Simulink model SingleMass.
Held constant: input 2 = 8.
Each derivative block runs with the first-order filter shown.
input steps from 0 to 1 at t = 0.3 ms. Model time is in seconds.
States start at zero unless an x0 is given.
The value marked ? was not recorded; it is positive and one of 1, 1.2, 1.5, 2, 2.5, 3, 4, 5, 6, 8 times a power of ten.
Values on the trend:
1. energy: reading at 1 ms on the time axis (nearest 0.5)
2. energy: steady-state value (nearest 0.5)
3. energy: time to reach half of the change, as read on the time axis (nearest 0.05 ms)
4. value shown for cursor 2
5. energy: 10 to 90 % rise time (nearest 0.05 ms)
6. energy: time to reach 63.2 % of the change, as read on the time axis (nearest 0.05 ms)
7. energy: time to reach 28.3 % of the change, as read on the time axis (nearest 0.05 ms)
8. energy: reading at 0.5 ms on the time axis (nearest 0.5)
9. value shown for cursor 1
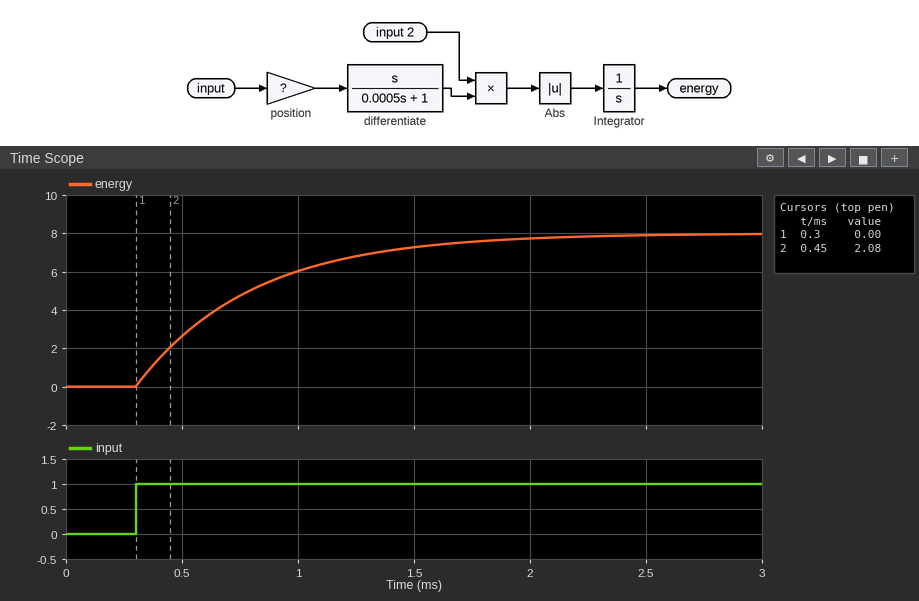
6.0
8.0
0.65 ms
2.08
1.10 ms
0.80 ms
0.45 ms
2.5
0.00
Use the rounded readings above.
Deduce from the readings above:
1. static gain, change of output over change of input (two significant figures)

8.0
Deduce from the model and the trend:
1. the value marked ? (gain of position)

1
